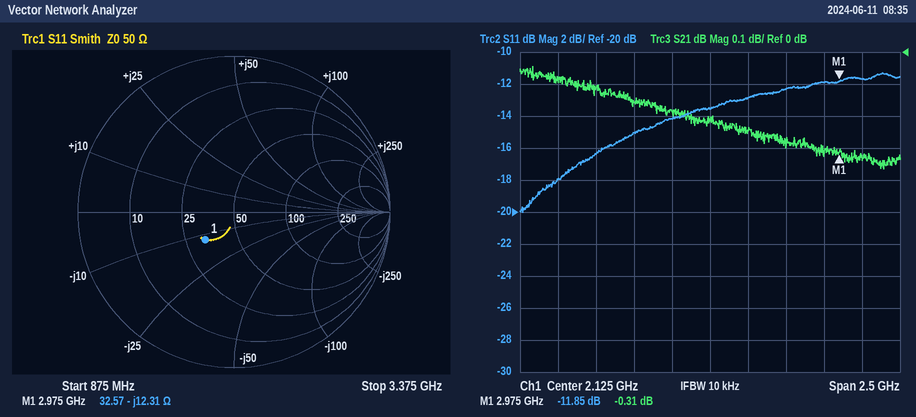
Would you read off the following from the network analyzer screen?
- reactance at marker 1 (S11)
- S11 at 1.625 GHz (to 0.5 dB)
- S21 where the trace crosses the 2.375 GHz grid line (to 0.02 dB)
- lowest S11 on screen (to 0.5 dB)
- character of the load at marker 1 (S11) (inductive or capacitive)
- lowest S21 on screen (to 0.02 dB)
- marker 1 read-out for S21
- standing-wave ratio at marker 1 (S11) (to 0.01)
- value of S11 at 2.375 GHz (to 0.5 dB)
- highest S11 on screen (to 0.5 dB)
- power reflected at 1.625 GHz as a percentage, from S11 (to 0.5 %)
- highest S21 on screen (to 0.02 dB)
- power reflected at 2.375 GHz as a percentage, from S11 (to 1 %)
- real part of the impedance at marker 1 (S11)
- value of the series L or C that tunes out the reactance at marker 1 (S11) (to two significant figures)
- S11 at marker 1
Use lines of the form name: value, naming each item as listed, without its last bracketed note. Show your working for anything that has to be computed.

reactance at marker 1: -12.31 Ω
S11 at 1.625 GHz: -15.0 dB
S21 where the trace crosses the 2.375 GHz grid line: -0.24 dB
lowest S11 on screen: -20.0 dB
character of the load at marker 1 (S11): capacitive
lowest S21 on screen: -0.36 dB
marker 1 read-out for S21: -0.31 dB
standing-wave ratio at marker 1 (S11): 1.69
value of S11 at 2.375 GHz: -13.0 dB
highest S11 on screen: -11.5 dB
power reflected at 1.625 GHz as a percentage, from S11: 10^(-15/10) ≈ 3.16 %, so 3.0 % to the nearest 0.5 %
highest S21 on screen: -0.04 dB
power reflected at 2.375 GHz as a percentage, from S11: 10^(-13/10) ≈ 5 %
real part of the impedance at marker 1: 32.57 Ω
value of the series L or C that tunes out the reactance at marker 1 (S11): L = 12.31 Ω/(2π × 2.975 GHz) ≈ 659 pH, so 660 pH to two significant figures
S11 at marker 1: -11.85 dB
